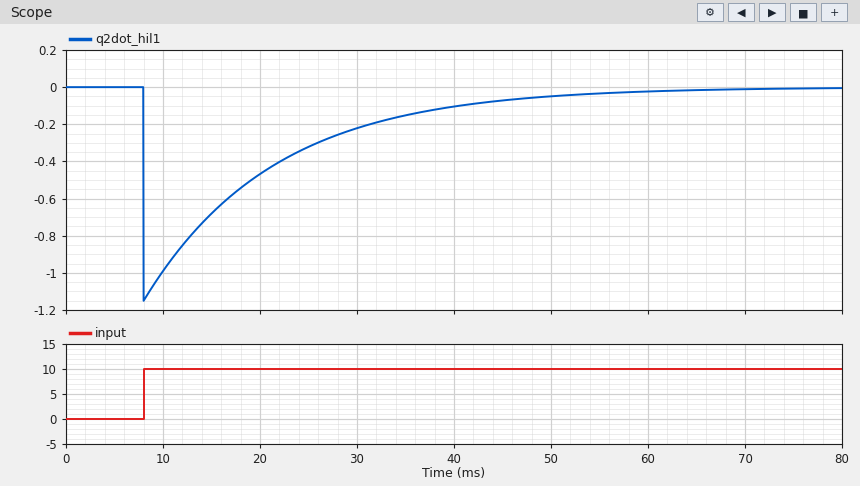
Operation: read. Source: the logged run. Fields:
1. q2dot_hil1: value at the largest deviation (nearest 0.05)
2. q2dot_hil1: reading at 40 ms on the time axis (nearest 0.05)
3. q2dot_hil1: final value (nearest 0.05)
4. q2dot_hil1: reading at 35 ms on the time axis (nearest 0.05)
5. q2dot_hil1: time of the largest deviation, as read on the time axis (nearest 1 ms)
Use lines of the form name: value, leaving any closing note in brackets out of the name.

q2dot_hil1: value at the largest deviation: -1.15
q2dot_hil1: reading at 40 ms on the time axis: -0.10
q2dot_hil1: final value: 0.00
q2dot_hil1: reading at 35 ms on the time axis: -0.15
q2dot_hil1: time of the largest deviation, as read on the time axis: 8 ms
